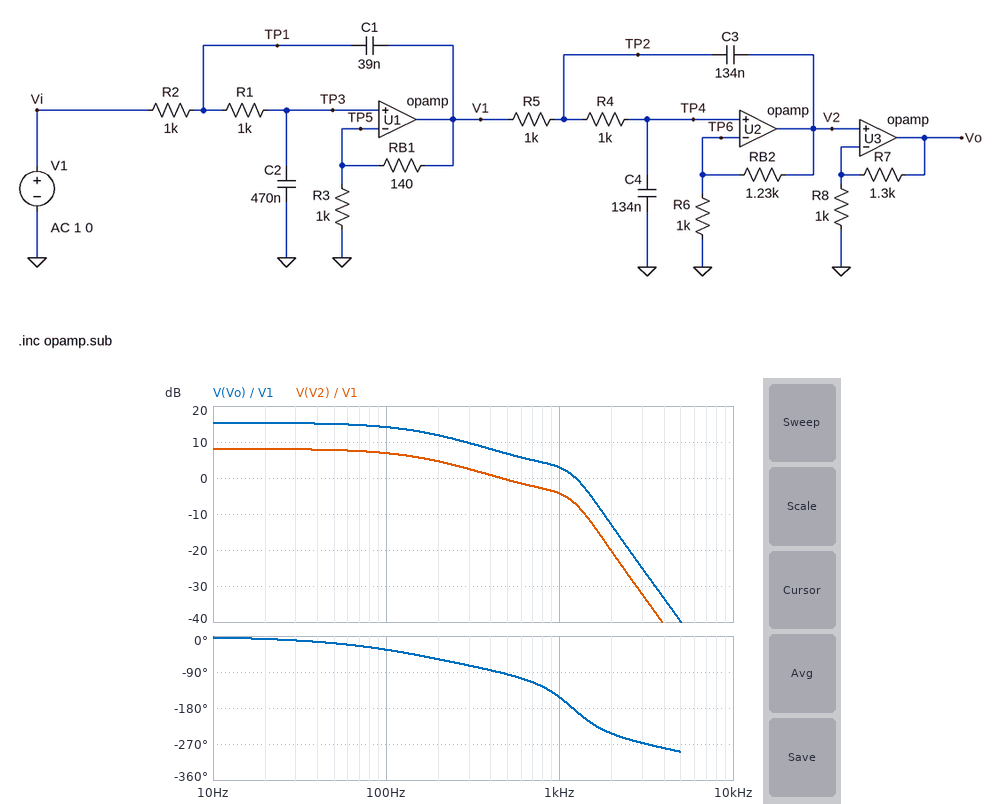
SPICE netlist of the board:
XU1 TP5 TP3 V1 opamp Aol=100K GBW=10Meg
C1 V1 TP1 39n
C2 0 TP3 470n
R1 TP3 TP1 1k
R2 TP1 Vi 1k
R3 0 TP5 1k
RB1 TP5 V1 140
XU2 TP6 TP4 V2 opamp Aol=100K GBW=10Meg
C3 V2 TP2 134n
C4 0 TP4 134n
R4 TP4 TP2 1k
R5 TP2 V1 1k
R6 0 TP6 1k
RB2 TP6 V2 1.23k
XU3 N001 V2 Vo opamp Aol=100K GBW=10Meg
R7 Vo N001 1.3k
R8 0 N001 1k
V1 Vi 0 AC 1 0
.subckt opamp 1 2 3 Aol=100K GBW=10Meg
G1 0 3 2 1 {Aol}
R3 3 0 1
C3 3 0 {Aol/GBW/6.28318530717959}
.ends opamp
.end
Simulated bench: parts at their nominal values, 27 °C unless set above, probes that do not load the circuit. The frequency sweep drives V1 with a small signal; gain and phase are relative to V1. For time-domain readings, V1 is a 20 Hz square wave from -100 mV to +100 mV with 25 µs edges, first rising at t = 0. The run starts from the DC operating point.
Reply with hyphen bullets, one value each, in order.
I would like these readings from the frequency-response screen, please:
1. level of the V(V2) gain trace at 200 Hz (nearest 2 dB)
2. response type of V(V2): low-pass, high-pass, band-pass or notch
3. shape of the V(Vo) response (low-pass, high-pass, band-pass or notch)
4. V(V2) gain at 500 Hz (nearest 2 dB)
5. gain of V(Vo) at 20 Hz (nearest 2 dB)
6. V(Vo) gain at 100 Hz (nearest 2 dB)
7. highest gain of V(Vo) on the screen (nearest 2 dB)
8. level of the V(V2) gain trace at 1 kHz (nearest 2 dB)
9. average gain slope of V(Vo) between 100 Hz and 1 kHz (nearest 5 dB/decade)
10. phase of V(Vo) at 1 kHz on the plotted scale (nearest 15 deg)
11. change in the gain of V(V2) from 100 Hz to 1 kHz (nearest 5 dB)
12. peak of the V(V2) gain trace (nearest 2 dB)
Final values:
- 4 dB
- low-pass
- low-pass
- 0 dB
- 16 dB
- 14 dB
- 16 dB
- -4 dB
- -10 dB/decade
- -150 deg
- -10 dB
- 8 dB
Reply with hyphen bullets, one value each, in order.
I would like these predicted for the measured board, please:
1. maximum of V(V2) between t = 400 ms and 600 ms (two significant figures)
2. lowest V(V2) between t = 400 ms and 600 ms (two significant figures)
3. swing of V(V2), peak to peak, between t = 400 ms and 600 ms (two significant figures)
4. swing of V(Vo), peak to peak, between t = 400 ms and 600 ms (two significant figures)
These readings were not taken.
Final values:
- 250 mV
- -250 mV
- 510 mV
- 1.2 V
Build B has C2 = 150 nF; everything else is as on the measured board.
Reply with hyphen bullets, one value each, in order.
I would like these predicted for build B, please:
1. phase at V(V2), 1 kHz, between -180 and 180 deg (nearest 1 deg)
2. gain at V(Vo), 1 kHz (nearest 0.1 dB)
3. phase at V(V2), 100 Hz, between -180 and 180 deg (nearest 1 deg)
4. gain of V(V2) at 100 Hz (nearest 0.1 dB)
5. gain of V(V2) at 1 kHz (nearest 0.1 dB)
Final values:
- -133 deg
- 12.3 dB
- -14 deg
- 8.0 dB
- 5.0 dB
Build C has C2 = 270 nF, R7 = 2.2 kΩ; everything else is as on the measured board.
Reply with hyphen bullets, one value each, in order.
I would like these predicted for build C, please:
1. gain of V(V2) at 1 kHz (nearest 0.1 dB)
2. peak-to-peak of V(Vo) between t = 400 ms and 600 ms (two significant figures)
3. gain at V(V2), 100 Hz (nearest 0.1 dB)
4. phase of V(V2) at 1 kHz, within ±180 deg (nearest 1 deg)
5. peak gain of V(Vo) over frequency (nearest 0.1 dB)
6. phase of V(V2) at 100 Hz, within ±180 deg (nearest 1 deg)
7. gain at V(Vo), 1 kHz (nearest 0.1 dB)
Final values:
- 0.4 dB
- 1.6 V
- 7.7 dB
- -146 deg
- 18.2 dB
- -22 deg
- 10.5 dB
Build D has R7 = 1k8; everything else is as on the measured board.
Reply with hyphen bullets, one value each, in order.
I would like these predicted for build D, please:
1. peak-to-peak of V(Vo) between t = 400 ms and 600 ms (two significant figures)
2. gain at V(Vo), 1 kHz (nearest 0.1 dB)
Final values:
- 1.4 V
- 4.6 dB
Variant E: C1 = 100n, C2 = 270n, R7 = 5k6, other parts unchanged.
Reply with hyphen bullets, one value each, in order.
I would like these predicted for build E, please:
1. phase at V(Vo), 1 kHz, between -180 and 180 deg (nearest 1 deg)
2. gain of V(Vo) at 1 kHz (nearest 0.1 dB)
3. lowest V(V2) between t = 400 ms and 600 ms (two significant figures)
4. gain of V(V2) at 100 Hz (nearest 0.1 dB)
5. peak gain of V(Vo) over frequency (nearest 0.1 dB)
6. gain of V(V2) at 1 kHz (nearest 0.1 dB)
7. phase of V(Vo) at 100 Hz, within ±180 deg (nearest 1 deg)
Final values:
- -157 deg
- 17.1 dB
- -250 mV
- 7.8 dB
- 24.5 dB
- 0.7 dB
- -22 deg
